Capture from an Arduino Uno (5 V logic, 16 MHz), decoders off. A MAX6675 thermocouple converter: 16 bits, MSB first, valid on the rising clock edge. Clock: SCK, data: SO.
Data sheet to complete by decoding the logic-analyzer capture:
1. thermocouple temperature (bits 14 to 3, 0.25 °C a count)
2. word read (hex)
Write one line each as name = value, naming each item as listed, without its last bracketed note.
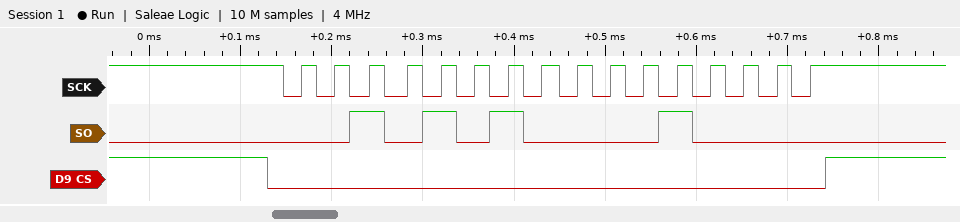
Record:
thermocouple temperature = 336.50 °C
word read = 0x2A10
